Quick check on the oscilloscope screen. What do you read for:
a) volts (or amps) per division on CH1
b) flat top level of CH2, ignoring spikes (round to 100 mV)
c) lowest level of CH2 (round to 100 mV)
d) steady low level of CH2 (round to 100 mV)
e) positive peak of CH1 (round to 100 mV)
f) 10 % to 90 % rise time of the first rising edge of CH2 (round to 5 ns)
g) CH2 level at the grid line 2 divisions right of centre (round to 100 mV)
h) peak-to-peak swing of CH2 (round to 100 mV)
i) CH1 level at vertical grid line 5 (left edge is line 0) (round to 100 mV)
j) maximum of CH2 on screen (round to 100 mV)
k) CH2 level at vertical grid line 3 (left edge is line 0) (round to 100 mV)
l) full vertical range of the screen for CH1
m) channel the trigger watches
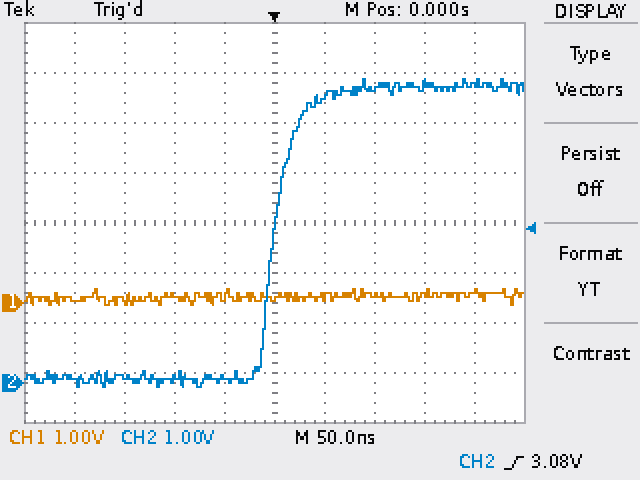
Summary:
1 V
5.9 V
-100 mV
100 mV
300 mV
40 ns
5.9 V
6.2 V
100 mV
6.1 V
100 mV
8 V
CH2
